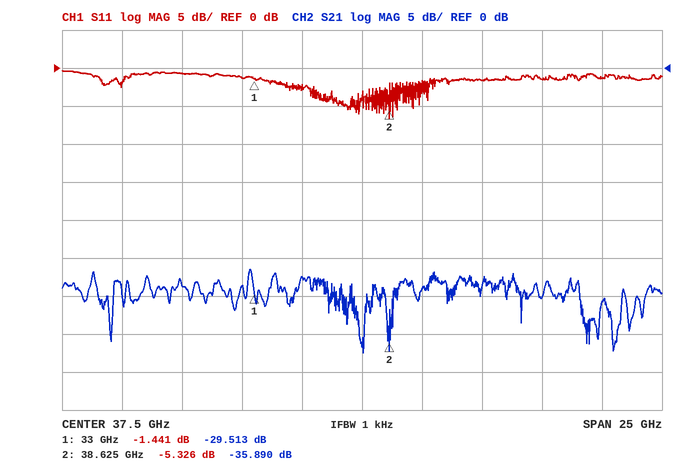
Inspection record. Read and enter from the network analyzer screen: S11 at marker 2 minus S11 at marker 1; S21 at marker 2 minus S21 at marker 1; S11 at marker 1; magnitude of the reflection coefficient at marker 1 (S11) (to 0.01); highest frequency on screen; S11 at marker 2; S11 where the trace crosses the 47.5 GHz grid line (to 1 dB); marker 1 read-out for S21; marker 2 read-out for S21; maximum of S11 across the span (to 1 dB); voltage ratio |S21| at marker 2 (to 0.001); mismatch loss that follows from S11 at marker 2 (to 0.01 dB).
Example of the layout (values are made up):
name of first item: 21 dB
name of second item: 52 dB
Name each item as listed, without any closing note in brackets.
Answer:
S11 at marker 2 minus S11 at marker 1: -3.885 dB
S21 at marker 2 minus S21 at marker 1: -6.377 dB
S11 at marker 1: -1.441 dB
magnitude of the reflection coefficient at marker 1 (S11): 0.85
highest frequency on screen: 50 GHz
S11 at marker 2: -5.326 dB
S11 where the trace crosses the 47.5 GHz grid line: -1 dB
marker 1 read-out for S21: -29.513 dB
marker 2 read-out for S21: -35.890 dB
maximum of S11 across the span: 0 dB
voltage ratio |S21| at marker 2: 0.016
mismatch loss that follows from S11 at marker 2: 1.51 dB
